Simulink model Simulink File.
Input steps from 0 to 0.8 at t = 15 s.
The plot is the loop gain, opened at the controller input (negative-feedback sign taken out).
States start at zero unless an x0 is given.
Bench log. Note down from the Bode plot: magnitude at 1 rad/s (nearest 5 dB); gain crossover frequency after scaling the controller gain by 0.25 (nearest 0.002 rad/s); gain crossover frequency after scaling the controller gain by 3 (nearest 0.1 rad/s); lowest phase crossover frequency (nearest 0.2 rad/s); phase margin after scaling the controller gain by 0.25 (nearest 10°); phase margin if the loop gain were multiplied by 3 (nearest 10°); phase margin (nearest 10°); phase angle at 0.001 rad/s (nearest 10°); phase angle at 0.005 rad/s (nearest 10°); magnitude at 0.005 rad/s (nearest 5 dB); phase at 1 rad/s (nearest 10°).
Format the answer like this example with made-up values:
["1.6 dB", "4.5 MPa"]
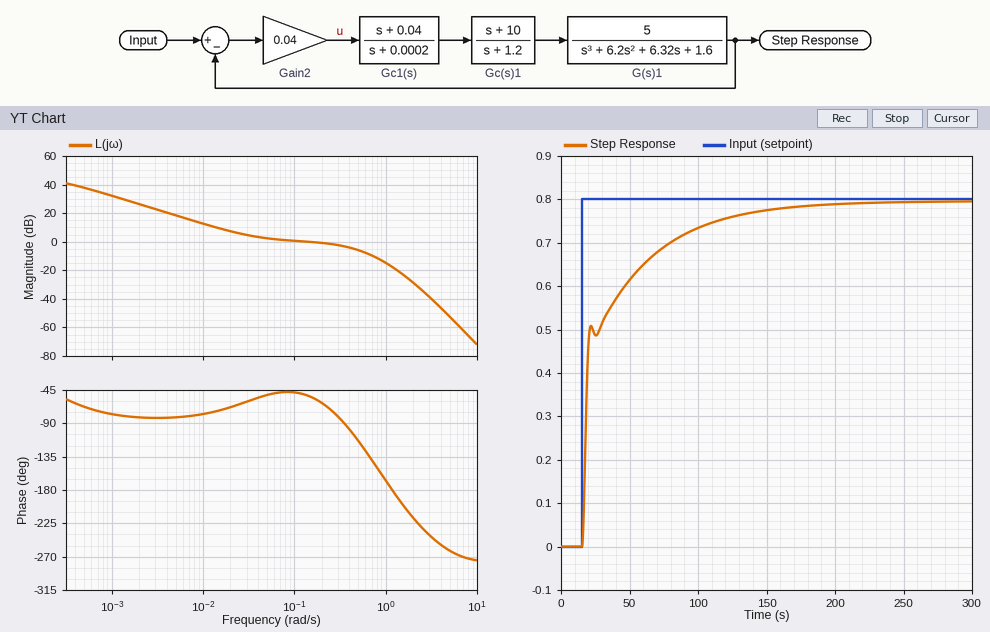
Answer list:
["-15 dB", "0.010 rad/s", "0.7 rad/s", "1.2 rad/s", "100°", "40°", "130°", "-80°", "-80°", "20 dB", "-170°"]
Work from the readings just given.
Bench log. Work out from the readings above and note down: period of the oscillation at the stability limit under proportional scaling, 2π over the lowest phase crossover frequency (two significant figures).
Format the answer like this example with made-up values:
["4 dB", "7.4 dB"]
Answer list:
["5.2 s"]
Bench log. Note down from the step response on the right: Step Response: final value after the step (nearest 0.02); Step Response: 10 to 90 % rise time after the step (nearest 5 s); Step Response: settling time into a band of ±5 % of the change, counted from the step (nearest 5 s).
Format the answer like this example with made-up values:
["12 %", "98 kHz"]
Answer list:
["0.80", "70 s", "105 s"]
